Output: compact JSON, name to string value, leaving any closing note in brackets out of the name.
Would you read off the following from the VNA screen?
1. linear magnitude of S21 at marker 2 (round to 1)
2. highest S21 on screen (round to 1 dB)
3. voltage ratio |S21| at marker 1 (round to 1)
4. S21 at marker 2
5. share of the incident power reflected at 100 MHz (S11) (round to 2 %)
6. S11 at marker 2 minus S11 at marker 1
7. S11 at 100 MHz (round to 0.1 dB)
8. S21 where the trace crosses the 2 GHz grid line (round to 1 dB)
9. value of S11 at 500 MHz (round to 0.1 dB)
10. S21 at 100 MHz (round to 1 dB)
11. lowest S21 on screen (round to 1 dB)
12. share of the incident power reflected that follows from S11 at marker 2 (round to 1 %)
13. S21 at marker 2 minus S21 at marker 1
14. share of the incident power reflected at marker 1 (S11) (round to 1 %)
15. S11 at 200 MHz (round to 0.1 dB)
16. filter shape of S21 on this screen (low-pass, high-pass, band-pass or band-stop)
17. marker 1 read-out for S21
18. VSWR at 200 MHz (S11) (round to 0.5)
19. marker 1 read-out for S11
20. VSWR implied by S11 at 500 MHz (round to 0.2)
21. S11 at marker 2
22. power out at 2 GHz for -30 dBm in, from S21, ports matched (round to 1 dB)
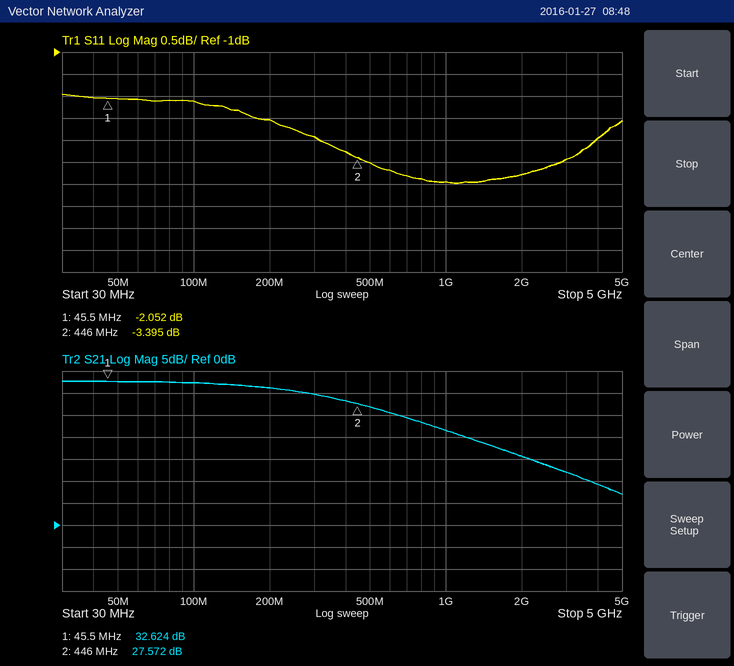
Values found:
{"linear magnitude of S21 at marker 2": "24", "highest S21 on screen": "33 dB", "voltage ratio |S21| at marker 1": "43", "S21 at marker 2": "27.572 dB", "share of the incident power reflected at 100 MHz (S11)": "62 %", "S11 at marker 2 minus S11 at marker 1": "-1.343 dB", "S11 at 100 MHz": "-2.1 dB", "S21 where the trace crosses the 2 GHz grid line": "16 dB", "value of S11 at 500 MHz": "-3.5 dB", "S21 at 100 MHz": "32 dB", "lowest S21 on screen": "7 dB", "share of the incident power reflected that follows from S11 at marker 2": "46 %", "S21 at marker 2 minus S21 at marker 1": "-5.052 dB", "share of the incident power reflected at marker 1 (S11)": "62 %", "S11 at 200 MHz": "-2.5 dB", "filter shape of S21 on this screen": "low-pass", "marker 1 read-out for S21": "32.624 dB", "VSWR at 200 MHz (S11)": "7.0", "marker 1 read-out for S11": "-2.052 dB", "VSWR implied by S11 at 500 MHz": "5.0", "S11 at marker 2": "-3.395 dB", "power out at 2 GHz for -30 dBm in, from S21, ports matched": "-14 dBm"}
